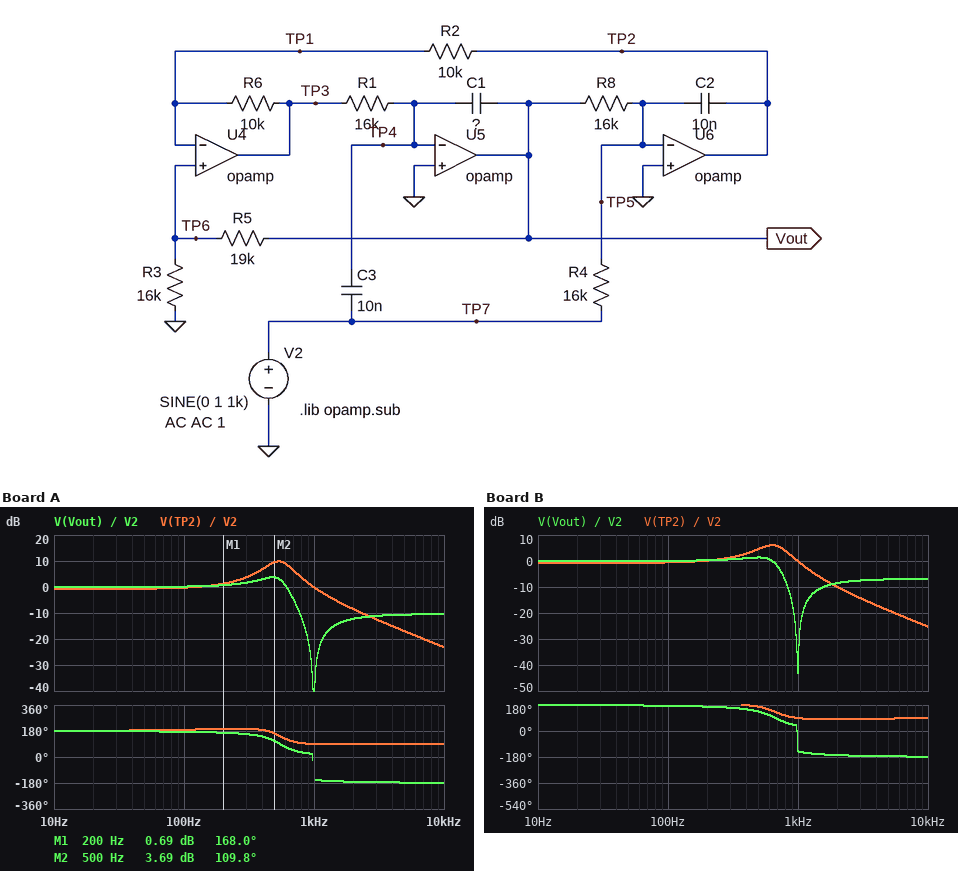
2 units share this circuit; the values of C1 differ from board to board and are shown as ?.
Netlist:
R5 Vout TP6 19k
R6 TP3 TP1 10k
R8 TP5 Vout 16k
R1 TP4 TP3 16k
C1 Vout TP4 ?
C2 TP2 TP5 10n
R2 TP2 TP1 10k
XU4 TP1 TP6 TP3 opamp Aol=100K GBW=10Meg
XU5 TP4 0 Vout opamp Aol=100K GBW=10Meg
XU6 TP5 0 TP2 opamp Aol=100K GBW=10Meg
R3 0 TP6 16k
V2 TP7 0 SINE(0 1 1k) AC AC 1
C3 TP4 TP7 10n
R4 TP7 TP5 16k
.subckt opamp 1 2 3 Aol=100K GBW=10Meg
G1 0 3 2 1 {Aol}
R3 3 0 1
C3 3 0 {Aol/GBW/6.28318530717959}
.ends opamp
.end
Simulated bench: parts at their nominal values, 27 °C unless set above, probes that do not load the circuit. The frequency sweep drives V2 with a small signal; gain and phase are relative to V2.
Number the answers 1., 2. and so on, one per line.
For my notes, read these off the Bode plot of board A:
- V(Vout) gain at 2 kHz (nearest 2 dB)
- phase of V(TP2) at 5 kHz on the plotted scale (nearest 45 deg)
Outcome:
1. -12 dB
2. 90 deg
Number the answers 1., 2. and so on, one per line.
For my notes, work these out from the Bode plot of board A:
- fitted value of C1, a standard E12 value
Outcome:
1. 33 nF
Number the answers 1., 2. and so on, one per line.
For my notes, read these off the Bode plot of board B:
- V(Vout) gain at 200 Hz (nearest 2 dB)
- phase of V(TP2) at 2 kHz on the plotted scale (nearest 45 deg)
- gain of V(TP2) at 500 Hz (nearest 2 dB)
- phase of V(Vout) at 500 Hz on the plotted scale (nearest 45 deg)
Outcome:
1. 0 dB
2. 90 deg
3. 4 dB
4. 135 deg
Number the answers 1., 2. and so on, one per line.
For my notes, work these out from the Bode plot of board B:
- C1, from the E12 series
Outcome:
1. 22 nF
